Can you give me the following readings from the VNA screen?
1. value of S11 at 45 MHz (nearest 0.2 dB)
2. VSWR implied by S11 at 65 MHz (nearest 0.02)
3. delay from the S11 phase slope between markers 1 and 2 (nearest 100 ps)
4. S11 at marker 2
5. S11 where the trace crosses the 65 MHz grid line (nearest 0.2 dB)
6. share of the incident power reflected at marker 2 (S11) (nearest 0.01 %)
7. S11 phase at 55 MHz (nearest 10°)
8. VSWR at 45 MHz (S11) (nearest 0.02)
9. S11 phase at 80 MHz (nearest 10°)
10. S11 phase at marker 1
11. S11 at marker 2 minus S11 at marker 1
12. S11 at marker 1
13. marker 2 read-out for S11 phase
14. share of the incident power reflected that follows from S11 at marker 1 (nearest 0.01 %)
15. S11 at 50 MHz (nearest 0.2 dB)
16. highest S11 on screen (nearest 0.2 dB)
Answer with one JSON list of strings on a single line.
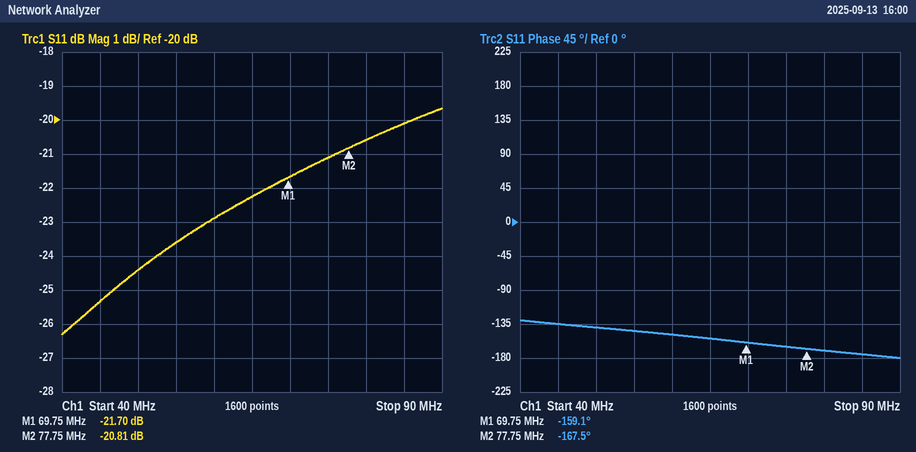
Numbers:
["-25.4 dB", "1.16", "2.9 ns", "-20.81 dB", "-22.2 dB", "0.83 %", "-140°", "1.12", "-170°", "-159.1°", "0.89 dB", "-21.70 dB", "-167.5°", "0.68 %", "-24.4 dB", "-19.6 dB"]
